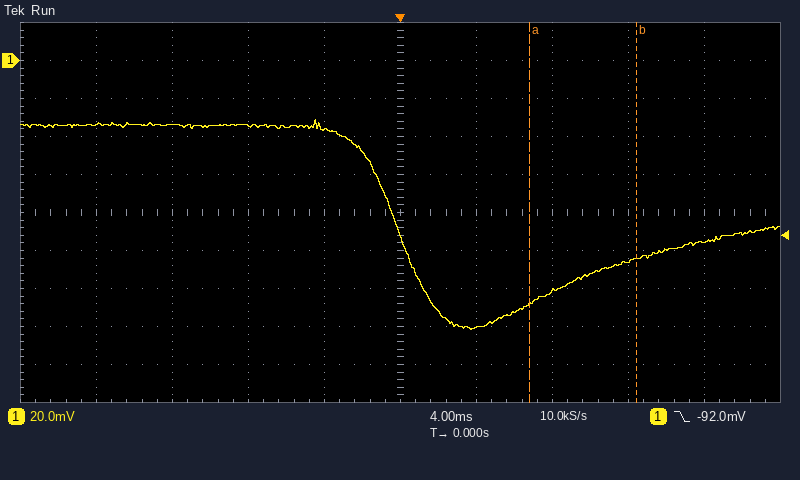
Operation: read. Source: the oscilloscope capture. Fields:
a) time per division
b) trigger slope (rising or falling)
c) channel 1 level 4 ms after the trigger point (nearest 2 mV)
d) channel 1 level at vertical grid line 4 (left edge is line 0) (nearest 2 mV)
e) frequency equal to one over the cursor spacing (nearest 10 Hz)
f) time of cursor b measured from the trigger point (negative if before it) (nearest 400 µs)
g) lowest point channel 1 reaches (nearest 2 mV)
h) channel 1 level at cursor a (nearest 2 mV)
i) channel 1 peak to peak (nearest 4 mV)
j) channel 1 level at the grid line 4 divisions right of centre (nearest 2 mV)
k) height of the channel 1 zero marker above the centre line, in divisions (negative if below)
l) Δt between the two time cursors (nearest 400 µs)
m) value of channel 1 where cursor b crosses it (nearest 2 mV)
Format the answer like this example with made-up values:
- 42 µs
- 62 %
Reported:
- 4 ms
- falling
- -140 mV
- -36 mV
- 180 Hz
- +12.4 ms
- -142 mV
- -128 mV
- 112 mV
- -96 mV
- +4.0 div
- 5.6 ms
- -104 mV
